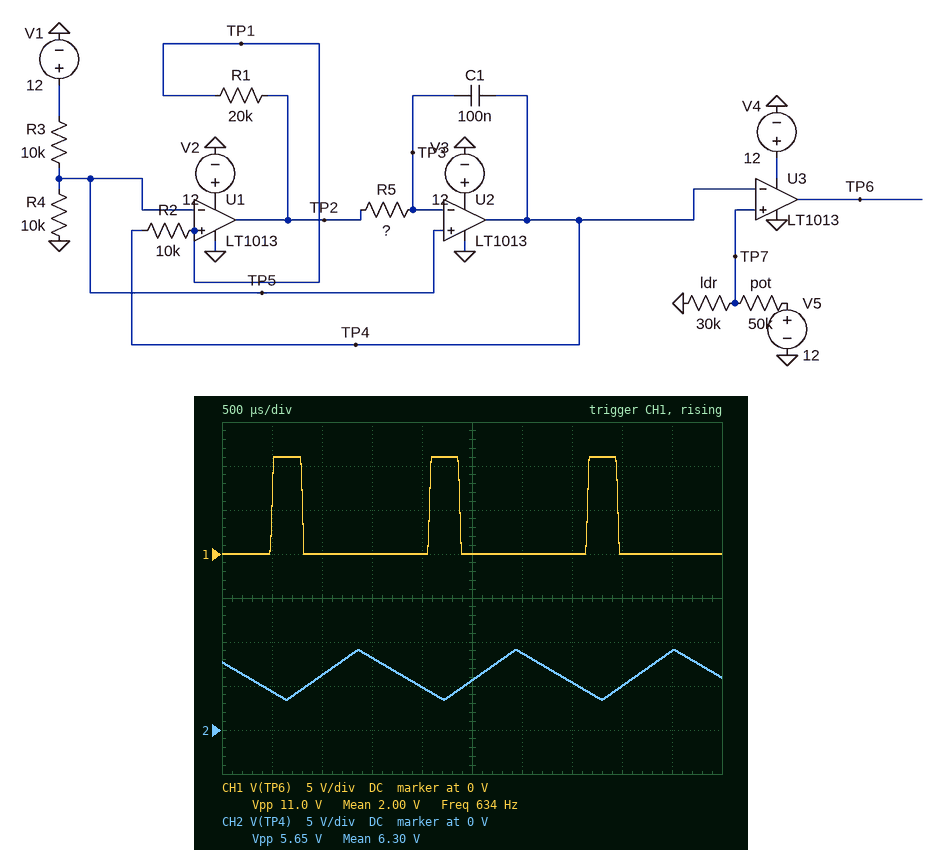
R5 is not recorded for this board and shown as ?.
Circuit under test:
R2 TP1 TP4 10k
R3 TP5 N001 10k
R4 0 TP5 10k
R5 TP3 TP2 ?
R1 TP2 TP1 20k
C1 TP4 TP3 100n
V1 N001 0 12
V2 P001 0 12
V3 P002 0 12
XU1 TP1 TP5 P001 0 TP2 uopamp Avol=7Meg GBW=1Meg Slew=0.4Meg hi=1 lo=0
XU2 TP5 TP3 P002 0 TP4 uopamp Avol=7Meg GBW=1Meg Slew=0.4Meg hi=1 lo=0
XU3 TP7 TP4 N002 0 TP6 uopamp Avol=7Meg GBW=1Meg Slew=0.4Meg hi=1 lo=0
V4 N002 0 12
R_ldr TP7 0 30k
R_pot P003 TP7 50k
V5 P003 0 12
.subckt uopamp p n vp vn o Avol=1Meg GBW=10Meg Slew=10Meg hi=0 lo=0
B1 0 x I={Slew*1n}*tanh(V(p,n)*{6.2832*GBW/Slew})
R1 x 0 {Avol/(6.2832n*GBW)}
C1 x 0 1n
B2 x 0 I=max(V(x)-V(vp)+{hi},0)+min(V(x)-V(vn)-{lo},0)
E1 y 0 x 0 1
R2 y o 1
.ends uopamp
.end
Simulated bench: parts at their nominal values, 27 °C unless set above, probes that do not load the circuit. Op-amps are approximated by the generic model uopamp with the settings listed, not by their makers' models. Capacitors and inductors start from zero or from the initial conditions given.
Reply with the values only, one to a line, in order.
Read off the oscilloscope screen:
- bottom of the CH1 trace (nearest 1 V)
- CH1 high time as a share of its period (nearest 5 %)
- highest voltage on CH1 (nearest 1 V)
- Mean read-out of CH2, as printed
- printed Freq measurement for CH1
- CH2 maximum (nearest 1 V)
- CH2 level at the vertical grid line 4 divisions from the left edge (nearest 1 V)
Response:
0 V
20 %
11 V
6.30 V
634 Hz
9 V
5 V
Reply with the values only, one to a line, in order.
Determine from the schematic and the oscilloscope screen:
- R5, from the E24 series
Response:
7.5 kΩ
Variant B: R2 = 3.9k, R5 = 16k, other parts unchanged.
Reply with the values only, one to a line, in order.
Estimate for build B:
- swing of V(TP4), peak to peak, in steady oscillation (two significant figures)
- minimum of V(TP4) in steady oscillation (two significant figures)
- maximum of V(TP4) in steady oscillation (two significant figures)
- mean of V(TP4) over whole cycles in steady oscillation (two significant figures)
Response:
2.2 V
5.0 V
7.2 V
6.1 V
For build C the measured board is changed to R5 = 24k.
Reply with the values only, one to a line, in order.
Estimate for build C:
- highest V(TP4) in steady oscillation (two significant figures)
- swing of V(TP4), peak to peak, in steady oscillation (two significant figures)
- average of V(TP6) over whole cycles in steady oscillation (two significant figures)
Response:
9.0 V
5.5 V
2.0 V
